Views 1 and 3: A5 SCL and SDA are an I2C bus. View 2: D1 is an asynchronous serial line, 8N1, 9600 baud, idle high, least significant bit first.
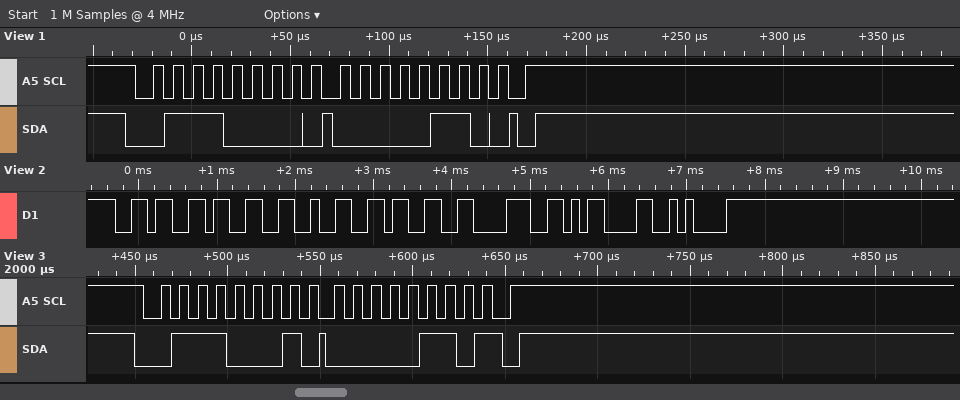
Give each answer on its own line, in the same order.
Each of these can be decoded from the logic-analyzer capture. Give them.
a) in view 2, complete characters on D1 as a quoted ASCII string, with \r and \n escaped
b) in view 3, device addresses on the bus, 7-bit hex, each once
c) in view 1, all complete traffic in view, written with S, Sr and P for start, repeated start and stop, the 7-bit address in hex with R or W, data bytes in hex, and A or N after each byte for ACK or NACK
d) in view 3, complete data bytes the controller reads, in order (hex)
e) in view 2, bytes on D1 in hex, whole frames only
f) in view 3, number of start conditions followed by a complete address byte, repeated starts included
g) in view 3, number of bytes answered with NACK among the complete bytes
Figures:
"63238\r\n"
0x38
S 38W A 06 A P
06
0x36 0x33 0x32 0x33 0x38 0x0D 0x0A
1
1
